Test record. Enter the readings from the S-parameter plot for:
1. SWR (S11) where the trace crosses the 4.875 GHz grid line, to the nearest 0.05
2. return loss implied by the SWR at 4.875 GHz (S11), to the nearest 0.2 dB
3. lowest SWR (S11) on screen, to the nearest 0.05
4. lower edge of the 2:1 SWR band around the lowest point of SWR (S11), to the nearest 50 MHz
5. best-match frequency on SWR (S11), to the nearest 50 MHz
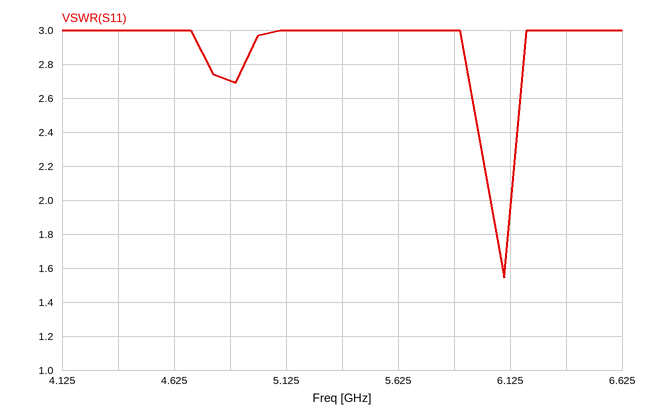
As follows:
2.70
6.8 dB
1.55
6.05 GHz
6.10 GHz
